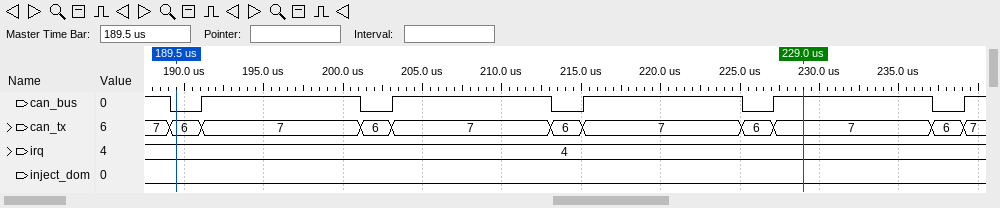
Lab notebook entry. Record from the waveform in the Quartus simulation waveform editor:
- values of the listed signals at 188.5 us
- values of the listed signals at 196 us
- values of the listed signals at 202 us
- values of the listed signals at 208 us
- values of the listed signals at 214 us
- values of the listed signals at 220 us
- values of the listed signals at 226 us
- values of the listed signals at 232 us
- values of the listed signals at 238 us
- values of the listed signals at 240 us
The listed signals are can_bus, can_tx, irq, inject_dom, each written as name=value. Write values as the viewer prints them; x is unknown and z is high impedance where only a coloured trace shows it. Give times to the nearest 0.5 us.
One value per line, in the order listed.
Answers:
can_bus=1, can_tx=7, irq=4, inject_dom=0
can_bus=1, can_tx=7, irq=4, inject_dom=0
can_bus=0, can_tx=6, irq=4, inject_dom=0
can_bus=1, can_tx=7, irq=4, inject_dom=0
can_bus=0, can_tx=6, irq=4, inject_dom=0
can_bus=1, can_tx=7, irq=4, inject_dom=0
can_bus=0, can_tx=6, irq=4, inject_dom=0
can_bus=1, can_tx=7, irq=4, inject_dom=0
can_bus=0, can_tx=6, irq=4, inject_dom=0
can_bus=1, can_tx=7, irq=4, inject_dom=0
